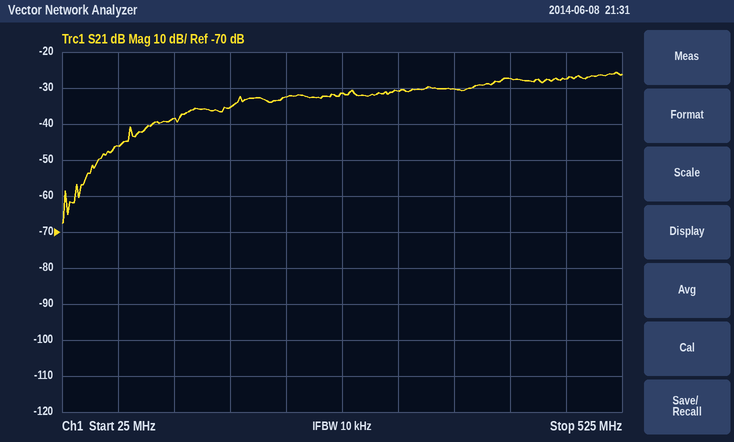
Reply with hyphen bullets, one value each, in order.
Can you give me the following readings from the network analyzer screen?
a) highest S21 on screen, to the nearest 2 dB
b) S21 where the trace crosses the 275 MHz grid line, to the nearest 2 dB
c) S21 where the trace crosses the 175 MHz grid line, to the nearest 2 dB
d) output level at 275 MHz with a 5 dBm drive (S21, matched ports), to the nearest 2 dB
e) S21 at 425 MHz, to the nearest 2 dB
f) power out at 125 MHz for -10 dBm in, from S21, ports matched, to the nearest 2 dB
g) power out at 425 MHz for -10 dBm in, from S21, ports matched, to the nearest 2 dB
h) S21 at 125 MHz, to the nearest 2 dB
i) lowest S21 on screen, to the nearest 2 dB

- -26 dB
- -32 dB
- -36 dB
- -26 dBm
- -28 dB
- -48 dBm
- -38 dBm
- -38 dB
- -68 dB
